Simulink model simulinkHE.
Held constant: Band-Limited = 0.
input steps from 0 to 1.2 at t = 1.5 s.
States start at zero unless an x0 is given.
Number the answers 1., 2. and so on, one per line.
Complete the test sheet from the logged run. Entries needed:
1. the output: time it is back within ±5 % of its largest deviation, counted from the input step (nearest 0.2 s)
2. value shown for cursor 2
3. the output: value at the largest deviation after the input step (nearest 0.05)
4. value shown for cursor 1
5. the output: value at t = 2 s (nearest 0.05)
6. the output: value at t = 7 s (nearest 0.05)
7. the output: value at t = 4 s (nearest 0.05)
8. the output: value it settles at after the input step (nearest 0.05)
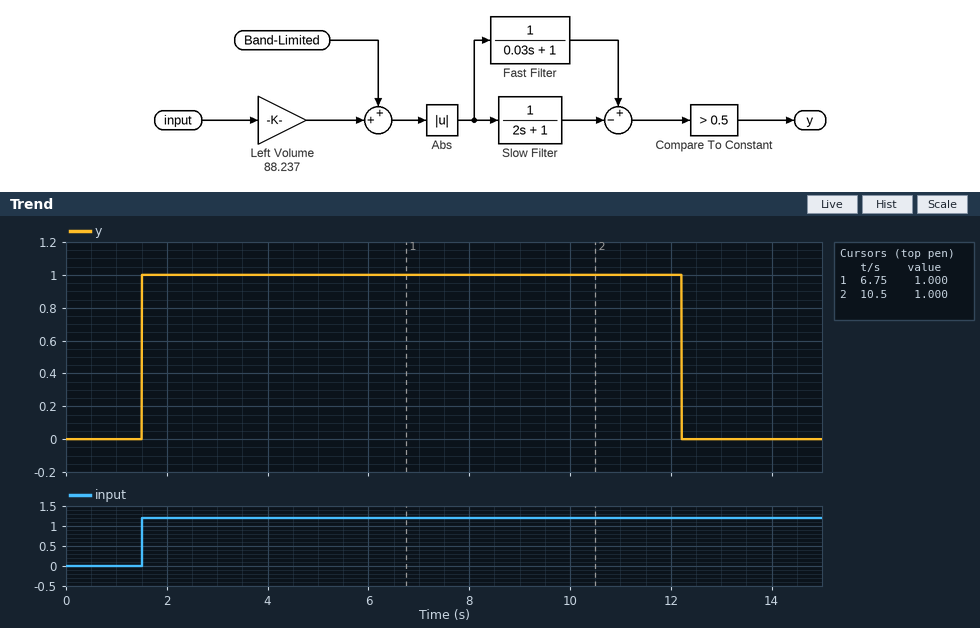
1. 10.8 s
2. 1.000
3. 1.00
4. 1.000
5. 1.00
6. 1.00
7. 1.00
8. 0.00
